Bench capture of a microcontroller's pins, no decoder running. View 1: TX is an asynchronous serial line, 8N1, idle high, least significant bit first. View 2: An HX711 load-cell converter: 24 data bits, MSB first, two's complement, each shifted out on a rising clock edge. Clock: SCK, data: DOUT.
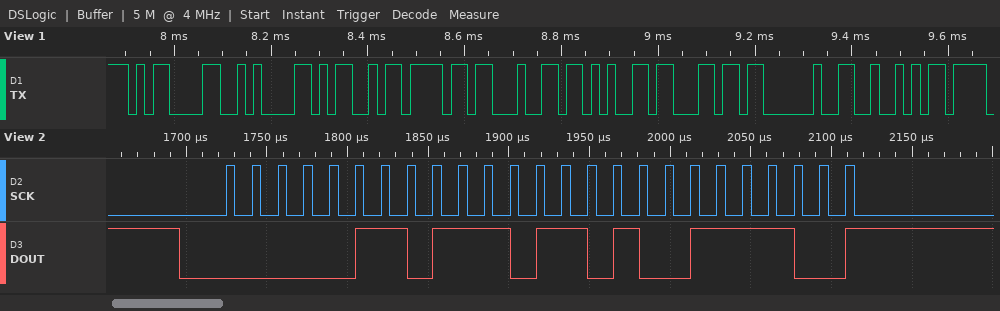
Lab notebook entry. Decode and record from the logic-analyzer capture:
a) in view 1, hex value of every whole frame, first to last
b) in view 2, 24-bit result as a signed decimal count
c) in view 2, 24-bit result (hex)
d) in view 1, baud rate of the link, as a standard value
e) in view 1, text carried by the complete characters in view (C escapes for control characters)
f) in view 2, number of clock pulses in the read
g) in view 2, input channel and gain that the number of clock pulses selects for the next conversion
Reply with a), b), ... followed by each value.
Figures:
a) 0D 0A 4D 6F 64 65 6C 20 52
b) 453948
c) 0x06ED3C
d) 57600 baud
e) "\r\nModel R"
f) 25
g) channel A, gain 128
